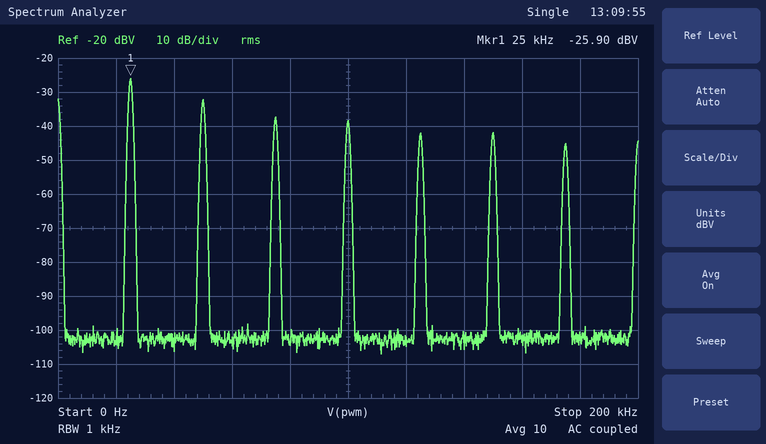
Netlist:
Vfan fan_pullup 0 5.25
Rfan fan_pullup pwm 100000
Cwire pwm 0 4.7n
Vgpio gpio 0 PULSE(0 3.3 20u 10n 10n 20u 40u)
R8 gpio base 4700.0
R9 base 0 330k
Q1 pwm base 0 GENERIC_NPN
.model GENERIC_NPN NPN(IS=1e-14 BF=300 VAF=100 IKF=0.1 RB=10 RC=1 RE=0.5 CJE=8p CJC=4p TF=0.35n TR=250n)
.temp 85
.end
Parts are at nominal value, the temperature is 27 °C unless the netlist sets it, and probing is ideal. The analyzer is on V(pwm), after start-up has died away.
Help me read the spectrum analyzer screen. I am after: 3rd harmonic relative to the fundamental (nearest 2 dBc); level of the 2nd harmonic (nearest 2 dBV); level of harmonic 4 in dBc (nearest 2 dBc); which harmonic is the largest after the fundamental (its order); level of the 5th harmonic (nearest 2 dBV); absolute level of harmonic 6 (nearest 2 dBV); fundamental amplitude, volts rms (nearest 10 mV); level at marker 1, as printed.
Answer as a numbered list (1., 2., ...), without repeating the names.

1. -12 dBc
2. -32 dBV
3. -12 dBc
4. 2
5. -42 dBV
6. -42 dBV
7. 50 mV
8. -25.90 dBV
